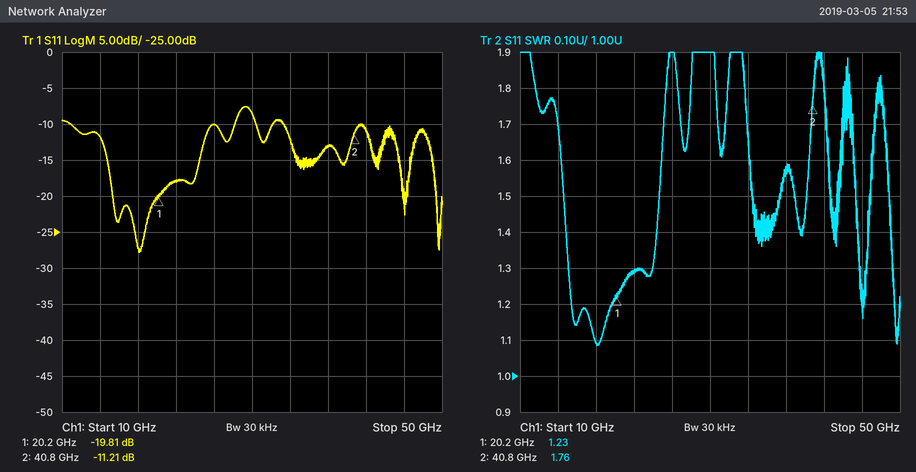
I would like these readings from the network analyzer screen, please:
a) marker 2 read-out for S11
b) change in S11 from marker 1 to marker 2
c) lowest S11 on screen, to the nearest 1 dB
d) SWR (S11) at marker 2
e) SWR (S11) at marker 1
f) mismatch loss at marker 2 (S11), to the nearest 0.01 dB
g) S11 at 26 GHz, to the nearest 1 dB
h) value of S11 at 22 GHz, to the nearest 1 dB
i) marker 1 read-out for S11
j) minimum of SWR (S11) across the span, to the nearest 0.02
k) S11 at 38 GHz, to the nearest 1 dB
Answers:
-11.21 dB
8.60 dB
-28 dB
1.76
1.23
0.34 dB
-10 dB
-18 dB
-19.81 dB
1.08
-13 dB
